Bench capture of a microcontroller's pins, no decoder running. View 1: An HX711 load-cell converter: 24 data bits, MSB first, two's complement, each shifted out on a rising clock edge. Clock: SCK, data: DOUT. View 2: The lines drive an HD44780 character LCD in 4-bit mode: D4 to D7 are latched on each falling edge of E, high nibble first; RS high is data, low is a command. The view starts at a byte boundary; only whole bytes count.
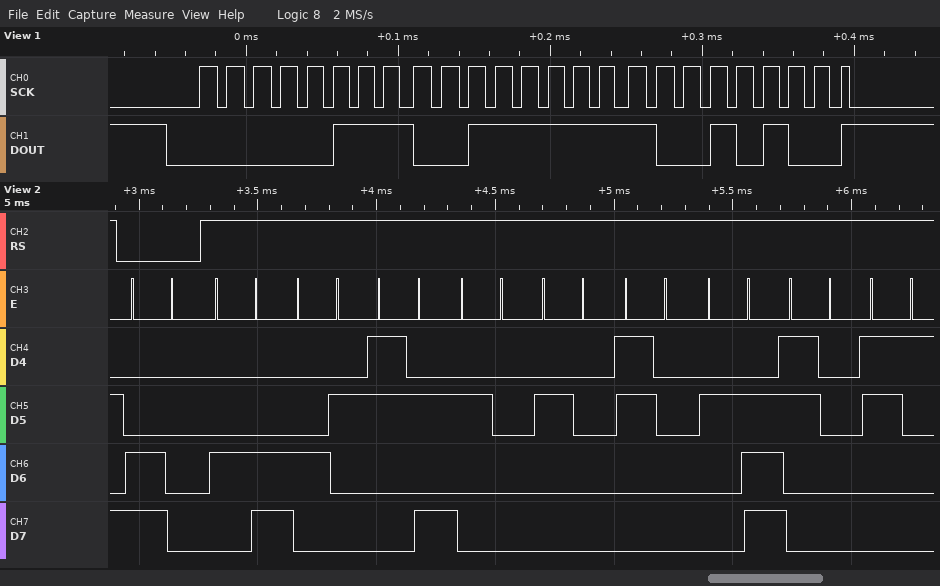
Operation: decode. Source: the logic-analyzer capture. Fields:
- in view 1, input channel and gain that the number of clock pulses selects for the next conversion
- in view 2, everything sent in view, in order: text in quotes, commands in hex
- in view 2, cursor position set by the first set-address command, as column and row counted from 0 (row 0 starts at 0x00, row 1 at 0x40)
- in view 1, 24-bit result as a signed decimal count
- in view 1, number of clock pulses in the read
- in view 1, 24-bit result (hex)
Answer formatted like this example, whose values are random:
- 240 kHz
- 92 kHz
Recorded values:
- channel A, gain 128
- 0xC0 "LB:  0.01"
- column 0, row 1
- 475028
- 25
- 0x073F94
